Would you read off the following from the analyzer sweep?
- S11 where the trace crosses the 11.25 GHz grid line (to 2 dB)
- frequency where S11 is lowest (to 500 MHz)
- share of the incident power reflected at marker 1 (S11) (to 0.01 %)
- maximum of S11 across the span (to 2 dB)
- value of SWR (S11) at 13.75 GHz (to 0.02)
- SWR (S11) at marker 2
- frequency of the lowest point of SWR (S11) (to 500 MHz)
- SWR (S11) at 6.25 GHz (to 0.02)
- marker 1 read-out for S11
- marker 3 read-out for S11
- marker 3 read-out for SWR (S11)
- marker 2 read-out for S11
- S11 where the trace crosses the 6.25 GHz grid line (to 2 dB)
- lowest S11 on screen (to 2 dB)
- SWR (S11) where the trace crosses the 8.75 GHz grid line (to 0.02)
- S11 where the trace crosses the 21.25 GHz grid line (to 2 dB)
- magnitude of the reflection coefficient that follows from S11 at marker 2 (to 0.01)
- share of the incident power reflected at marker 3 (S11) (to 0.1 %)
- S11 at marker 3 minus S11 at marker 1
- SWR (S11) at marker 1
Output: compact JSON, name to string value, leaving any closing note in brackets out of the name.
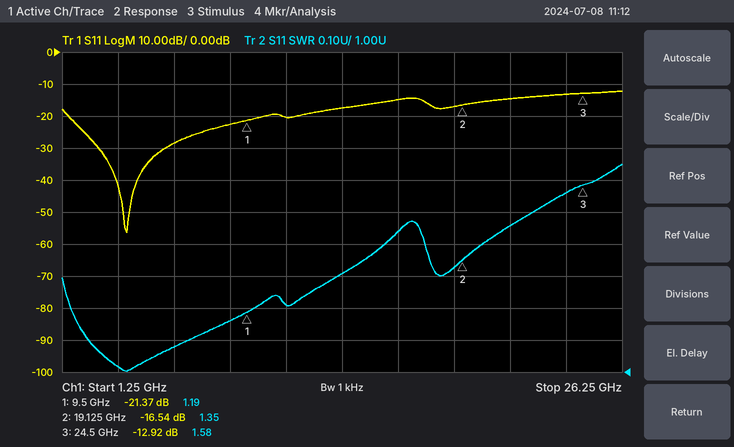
{"S11 where the trace crosses the 11.25 GHz grid line": "-20 dB", "frequency where S11 is lowest": "4.0 GHz", "share of the incident power reflected at marker 1 (S11)": "0.73 %", "maximum of S11 across the span": "-12 dB", "value of SWR (S11) at 13.75 GHz": "1.30", "SWR (S11) at marker 2": "1.35", "frequency of the lowest point of SWR (S11)": "4.0 GHz", "SWR (S11) at 6.25 GHz": "1.08", "marker 1 read-out for S11": "-21.37 dB", "marker 3 read-out for S11": "-12.92 dB", "marker 3 read-out for SWR": "1.58", "marker 2 read-out for S11": "-16.54 dB", "S11 where the trace crosses the 6.25 GHz grid line": "-28 dB", "lowest S11 on screen": "-56 dB", "SWR (S11) where the trace crosses the 8.75 GHz grid line": "1.16", "S11 where the trace crosses the 21.25 GHz grid line": "-14 dB", "magnitude of the reflection coefficient that follows from S11 at marker 2": "0.15", "share of the incident power reflected at marker 3 (S11)": "5.1 %", "S11 at marker 3 minus S11 at marker 1": "8.45 dB", "SWR (S11) at marker 1": "1.19"}
